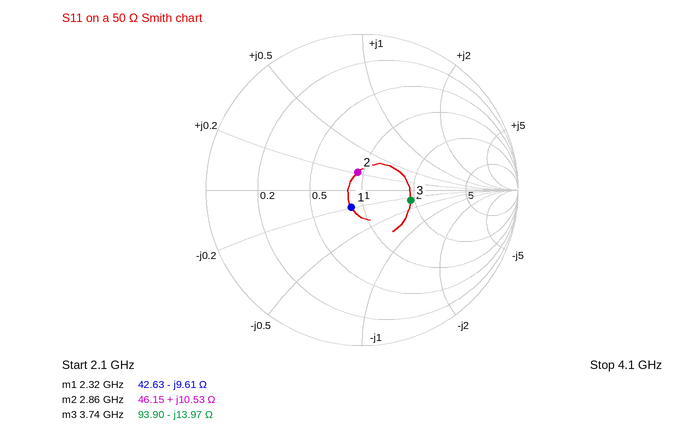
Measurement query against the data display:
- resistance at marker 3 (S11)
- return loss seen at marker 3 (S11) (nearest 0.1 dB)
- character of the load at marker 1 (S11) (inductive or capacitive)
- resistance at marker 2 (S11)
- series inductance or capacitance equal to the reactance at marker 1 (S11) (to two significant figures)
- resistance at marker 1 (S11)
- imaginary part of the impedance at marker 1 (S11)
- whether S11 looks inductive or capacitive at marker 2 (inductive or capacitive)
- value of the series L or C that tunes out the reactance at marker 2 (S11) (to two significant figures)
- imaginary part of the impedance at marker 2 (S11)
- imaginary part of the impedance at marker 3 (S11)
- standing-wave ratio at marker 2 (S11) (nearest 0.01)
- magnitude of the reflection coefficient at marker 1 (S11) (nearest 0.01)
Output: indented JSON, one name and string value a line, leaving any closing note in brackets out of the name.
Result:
{
  "resistance at marker 3": "93.90 Ω",
  "return loss seen at marker 3 (S11)": "9.9 dB",
  "character of the load at marker 1 (S11)": "capacitive",
  "resistance at marker 2": "46.15 Ω",
  "series inductance or capacitance equal to the reactance at marker 1 (S11)": "7.1 pF",
  "resistance at marker 1": "42.63 Ω",
  "imaginary part of the impedance at marker 1": "-9.61 Ω",
  "whether S11 looks inductive or capacitive at marker 2": "inductive",
  "value of the series L or C that tunes out the reactance at marker 2 (S11)": "5.3 pF",
  "imaginary part of the impedance at marker 2": "+10.53 Ω",
  "imaginary part of the impedance at marker 3": "-13.97 Ω",
  "standing-wave ratio at marker 2 (S11)": "1.26",
  "magnitude of the reflection coefficient at marker 1 (S11)": "0.13"
}
